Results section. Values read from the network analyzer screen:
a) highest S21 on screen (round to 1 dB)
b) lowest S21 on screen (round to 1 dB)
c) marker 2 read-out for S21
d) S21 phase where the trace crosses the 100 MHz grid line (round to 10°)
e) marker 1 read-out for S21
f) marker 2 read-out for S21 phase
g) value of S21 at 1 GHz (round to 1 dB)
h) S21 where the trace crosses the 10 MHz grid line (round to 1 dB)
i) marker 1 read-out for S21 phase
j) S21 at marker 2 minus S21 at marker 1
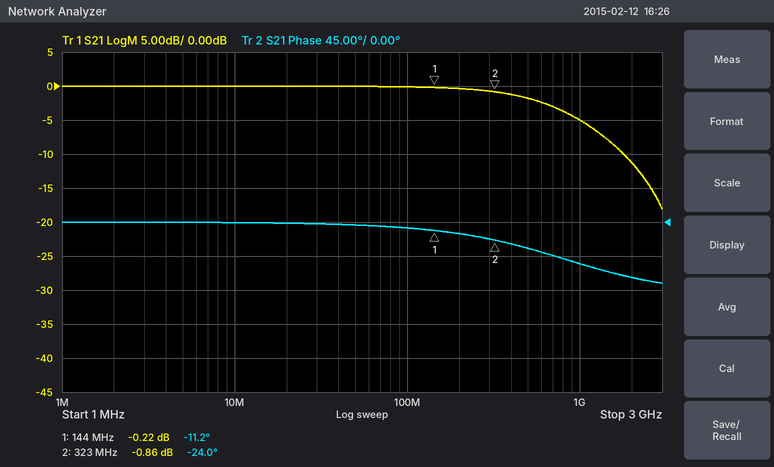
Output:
0 dB
-18 dB
-0.86 dB
-10°
-0.22 dB
-24.0°
-5 dB
0 dB
-11.2°
-0.64 dB
